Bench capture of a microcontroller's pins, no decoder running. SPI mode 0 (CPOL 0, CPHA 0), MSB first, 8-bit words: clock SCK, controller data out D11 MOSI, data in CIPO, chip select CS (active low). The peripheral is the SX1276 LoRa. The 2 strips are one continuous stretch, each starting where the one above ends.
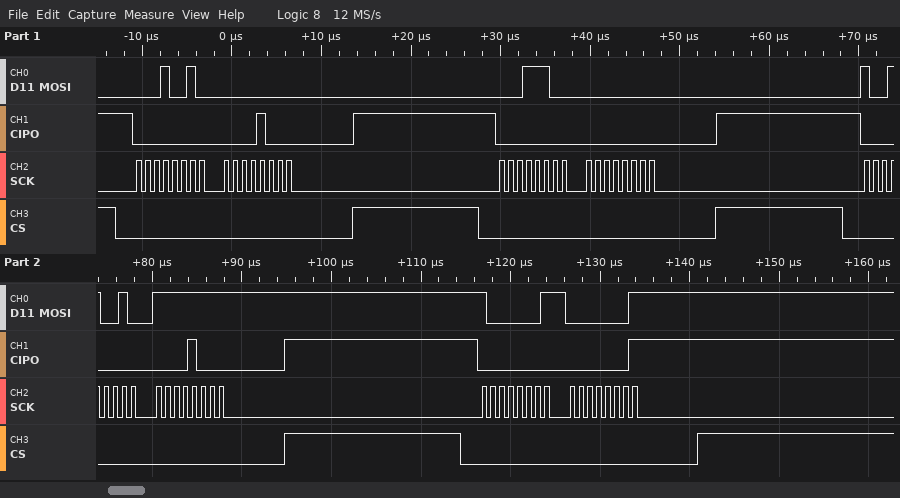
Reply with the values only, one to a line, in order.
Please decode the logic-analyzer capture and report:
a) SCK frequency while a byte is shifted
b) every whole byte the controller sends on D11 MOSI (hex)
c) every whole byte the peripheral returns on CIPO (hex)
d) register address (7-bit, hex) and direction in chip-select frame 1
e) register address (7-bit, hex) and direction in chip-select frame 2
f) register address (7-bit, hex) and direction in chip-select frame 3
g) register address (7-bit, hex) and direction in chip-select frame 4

1 MHz
12 00 1C 00 92 FF 81 01
00 08 00 00 00 08 00 01
0x12 read
0x1C read
0x12 write
0x01 write
